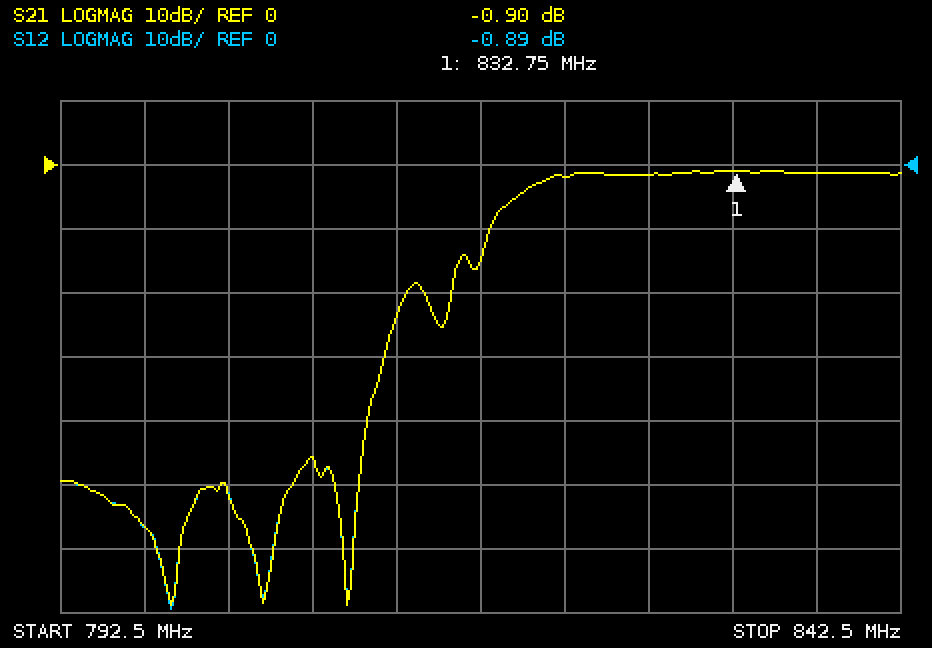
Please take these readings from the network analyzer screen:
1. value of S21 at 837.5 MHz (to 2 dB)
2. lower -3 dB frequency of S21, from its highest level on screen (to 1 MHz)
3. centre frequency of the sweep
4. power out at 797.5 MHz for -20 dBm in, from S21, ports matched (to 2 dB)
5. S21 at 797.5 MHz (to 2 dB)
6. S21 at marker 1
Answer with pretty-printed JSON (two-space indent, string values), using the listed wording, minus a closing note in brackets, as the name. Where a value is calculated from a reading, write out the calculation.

{
  "value of S21 at 837.5 MHz": "-2 dB",
  "lower -3 dB frequency of S21, from its highest level on screen": "820 MHz",
  "centre frequency of the sweep": "817.5 MHz",
  "power out at 797.5 MHz for -20 dBm in, from S21, ports matched": "-20 dBm + (-56 dB) = -76 dBm",
  "S21 at 797.5 MHz": "-56 dB",
  "S21 at marker 1": "-0.90 dB"
}
